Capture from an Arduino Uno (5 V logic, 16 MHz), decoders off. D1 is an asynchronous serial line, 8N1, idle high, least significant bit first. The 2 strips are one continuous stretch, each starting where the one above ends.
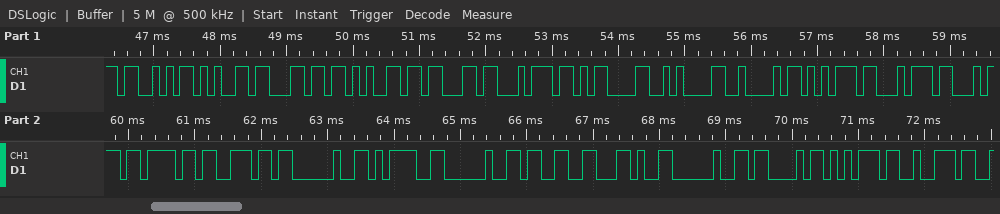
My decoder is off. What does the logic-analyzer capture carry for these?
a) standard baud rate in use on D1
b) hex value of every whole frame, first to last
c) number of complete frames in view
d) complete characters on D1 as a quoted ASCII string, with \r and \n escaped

9600 baud
0x53 0x65 0x6C 0x65 0x63 0x74 0x0D 0x0A 0x42 0x75 0x74 0x74 0x6F 0x6E 0x20 0x3D 0x20 0x33 0x2C 0x20 0x43 0x75 0x72
23
"Select\r\nButton = 3, Cur"
